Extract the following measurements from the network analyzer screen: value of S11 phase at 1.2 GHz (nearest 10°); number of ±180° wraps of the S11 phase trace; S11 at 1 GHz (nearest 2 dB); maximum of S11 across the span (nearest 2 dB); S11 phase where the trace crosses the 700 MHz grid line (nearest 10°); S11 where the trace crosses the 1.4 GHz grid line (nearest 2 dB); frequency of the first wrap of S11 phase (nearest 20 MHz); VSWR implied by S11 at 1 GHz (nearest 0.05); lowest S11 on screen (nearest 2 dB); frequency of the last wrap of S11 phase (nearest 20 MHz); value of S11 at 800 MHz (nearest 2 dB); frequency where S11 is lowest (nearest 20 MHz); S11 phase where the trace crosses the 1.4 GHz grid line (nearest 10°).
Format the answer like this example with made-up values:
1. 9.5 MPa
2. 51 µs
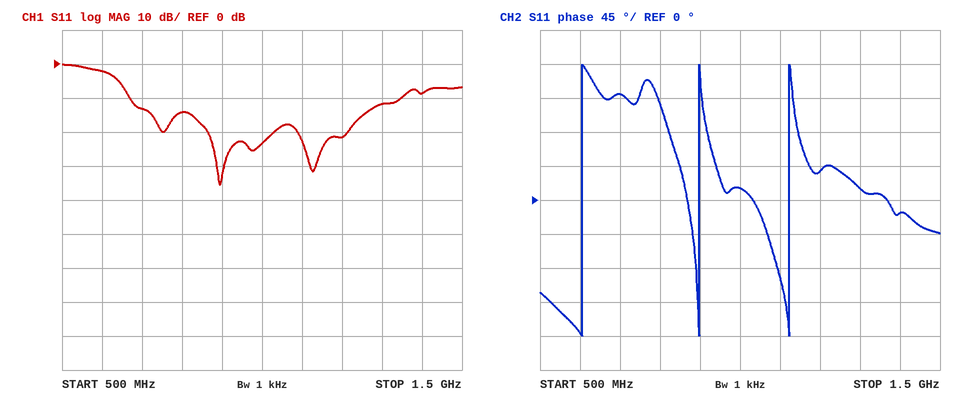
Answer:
1. 40°
2. 3
3. -24 dB
4. 0 dB
5. 140°
6. -8 dB
7. 600 MHz
8. 1.15
9. -36 dB
10. 1.12 GHz
11. -14 dB
12. 900 MHz
13. -20°
